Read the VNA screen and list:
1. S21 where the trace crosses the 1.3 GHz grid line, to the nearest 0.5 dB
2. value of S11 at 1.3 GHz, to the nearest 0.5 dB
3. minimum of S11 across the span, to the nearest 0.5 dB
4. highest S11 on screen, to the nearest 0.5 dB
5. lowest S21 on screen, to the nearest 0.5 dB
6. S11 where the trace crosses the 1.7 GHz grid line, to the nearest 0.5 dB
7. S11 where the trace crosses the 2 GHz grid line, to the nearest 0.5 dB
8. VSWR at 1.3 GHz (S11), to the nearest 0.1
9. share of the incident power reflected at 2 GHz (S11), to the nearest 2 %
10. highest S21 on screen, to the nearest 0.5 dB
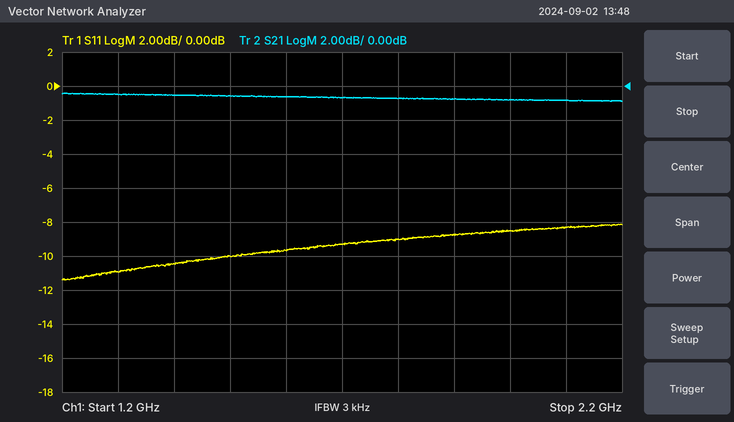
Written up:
-0.5 dB
-11.0 dB
-11.5 dB
-8.0 dB
-1.0 dB
-9.5 dB
-8.5 dB
1.8
14 %
-0.5 dB
